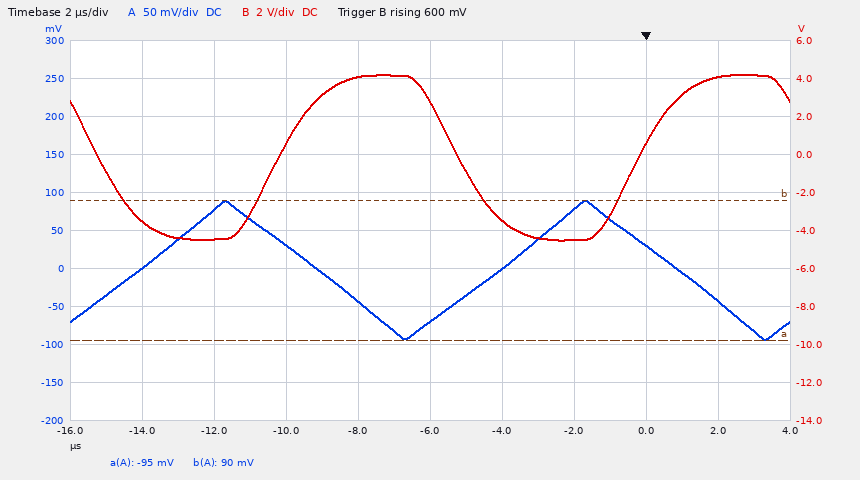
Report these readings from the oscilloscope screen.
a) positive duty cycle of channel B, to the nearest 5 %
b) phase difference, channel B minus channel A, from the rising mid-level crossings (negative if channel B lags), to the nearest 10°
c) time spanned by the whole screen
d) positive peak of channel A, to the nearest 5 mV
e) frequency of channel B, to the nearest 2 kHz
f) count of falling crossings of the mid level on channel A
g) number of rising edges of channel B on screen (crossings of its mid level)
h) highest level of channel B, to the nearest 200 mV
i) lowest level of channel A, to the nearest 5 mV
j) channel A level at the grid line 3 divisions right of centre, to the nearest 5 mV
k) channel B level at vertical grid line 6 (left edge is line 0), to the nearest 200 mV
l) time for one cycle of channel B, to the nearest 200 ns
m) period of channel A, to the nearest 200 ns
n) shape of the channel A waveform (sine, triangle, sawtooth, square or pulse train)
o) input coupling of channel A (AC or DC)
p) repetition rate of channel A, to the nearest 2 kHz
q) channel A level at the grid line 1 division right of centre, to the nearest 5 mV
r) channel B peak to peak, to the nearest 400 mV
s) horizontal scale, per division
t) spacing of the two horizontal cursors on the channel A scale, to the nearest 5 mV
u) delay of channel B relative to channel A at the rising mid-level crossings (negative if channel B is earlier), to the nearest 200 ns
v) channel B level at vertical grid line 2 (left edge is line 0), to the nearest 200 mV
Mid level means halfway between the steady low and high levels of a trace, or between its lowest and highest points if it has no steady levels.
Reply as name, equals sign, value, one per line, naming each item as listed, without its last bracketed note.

positive duty cycle of channel B, to the nearest 5 % = 50 %
phase difference, channel B minus channel A, from the rising mid-level crossings (negative if channel B lags), to the nearest 10° = -140°
time spanned by the whole screen = 20 µs
positive peak of channel A, to the nearest 5 mV = 90 mV
frequency of channel B, to the nearest 2 kHz = 100 kHz
count of falling crossings of the mid level on channel A = 2
number of rising edges of channel B on screen = 2
highest level of channel B, to the nearest 200 mV = 4.2 V
lowest level of channel A, to the nearest 5 mV = -95 mV
channel A level at the grid line 3 divisions right of centre, to the nearest 5 mV = 30 mV
channel B level at vertical grid line 6 (left edge is line 0), to the nearest 200 mV = -3.4 V
time for one cycle of channel B, to the nearest 200 ns = 10.0 µs
period of channel A, to the nearest 200 ns = 10.0 µs
shape of the channel A waveform = triangle
input coupling of channel A = DC
repetition rate of channel A, to the nearest 2 kHz = 100 kHz
channel A level at the grid line 1 division right of centre, to the nearest 5 mV = 0 mV
channel B peak to peak, to the nearest 400 mV = 8.8 V
horizontal scale, per division = 2 µs
spacing of the two horizontal cursors on the channel A scale, to the nearest 5 mV = 185 mV
delay of channel B relative to channel A at the rising mid-level crossings (negative if channel B is earlier), to the nearest 200 ns = +3.8 µs
channel B level at vertical grid line 2 (left edge is line 0), to the nearest 200 mV = -4.4 V
